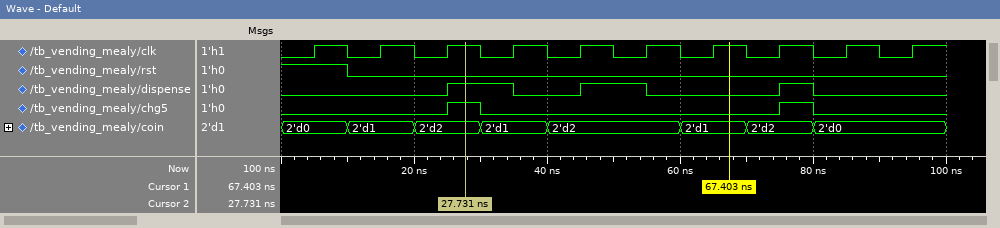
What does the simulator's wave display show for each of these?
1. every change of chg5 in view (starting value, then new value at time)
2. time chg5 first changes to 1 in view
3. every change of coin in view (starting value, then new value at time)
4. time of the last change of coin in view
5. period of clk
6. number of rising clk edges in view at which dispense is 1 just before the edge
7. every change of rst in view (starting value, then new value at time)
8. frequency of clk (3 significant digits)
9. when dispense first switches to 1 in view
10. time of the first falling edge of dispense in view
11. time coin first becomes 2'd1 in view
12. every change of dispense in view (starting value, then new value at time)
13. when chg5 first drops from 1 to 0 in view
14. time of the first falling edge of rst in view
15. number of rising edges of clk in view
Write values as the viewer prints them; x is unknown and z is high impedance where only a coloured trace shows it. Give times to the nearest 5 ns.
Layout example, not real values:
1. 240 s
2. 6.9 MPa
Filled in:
1. 0, 1 at 25 ns, 0 at 30 ns, 1 at 75 ns, 0 at 80 ns
2. 25 ns
3. 2'd0, 2'd1 at 10 ns, 2'd2 at 20 ns, 2'd1 at 30 ns, 2'd2 at 40 ns, 2'd1 at 60 ns, 2'd2 at 70 ns, 2'd0 at 80 ns
4. 80 ns
5. 10 ns
6. 2
7. 1, 0 at 10 ns
8. 100 MHz
9. 25 ns
10. 35 ns
11. 10 ns
12. 0, 1 at 25 ns, 0 at 35 ns, 1 at 45 ns, 0 at 55 ns, 1 at 75 ns, 0 at 80 ns
13. 30 ns
14. 10 ns
15. 10
